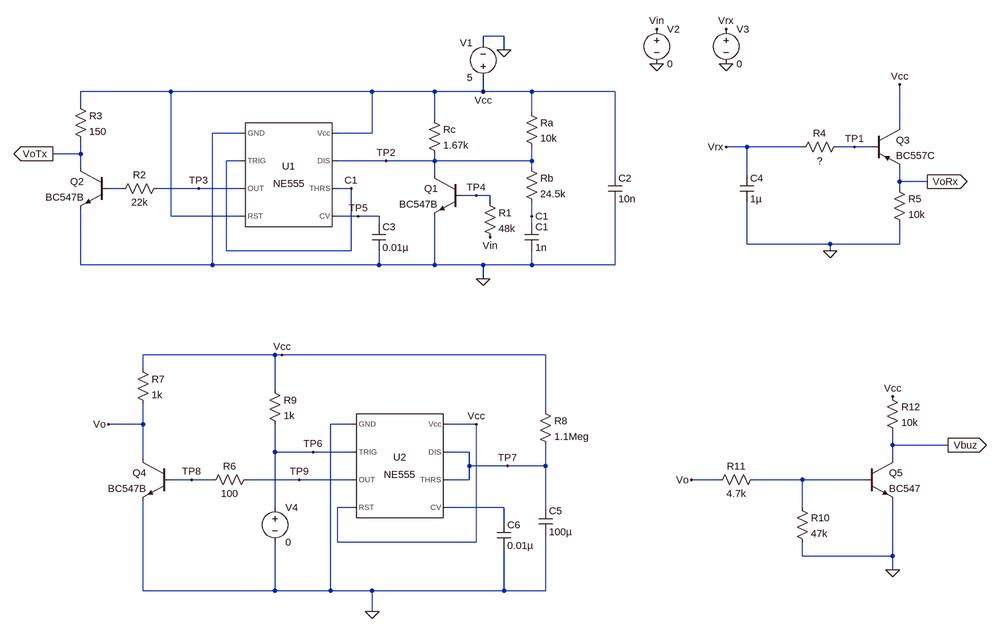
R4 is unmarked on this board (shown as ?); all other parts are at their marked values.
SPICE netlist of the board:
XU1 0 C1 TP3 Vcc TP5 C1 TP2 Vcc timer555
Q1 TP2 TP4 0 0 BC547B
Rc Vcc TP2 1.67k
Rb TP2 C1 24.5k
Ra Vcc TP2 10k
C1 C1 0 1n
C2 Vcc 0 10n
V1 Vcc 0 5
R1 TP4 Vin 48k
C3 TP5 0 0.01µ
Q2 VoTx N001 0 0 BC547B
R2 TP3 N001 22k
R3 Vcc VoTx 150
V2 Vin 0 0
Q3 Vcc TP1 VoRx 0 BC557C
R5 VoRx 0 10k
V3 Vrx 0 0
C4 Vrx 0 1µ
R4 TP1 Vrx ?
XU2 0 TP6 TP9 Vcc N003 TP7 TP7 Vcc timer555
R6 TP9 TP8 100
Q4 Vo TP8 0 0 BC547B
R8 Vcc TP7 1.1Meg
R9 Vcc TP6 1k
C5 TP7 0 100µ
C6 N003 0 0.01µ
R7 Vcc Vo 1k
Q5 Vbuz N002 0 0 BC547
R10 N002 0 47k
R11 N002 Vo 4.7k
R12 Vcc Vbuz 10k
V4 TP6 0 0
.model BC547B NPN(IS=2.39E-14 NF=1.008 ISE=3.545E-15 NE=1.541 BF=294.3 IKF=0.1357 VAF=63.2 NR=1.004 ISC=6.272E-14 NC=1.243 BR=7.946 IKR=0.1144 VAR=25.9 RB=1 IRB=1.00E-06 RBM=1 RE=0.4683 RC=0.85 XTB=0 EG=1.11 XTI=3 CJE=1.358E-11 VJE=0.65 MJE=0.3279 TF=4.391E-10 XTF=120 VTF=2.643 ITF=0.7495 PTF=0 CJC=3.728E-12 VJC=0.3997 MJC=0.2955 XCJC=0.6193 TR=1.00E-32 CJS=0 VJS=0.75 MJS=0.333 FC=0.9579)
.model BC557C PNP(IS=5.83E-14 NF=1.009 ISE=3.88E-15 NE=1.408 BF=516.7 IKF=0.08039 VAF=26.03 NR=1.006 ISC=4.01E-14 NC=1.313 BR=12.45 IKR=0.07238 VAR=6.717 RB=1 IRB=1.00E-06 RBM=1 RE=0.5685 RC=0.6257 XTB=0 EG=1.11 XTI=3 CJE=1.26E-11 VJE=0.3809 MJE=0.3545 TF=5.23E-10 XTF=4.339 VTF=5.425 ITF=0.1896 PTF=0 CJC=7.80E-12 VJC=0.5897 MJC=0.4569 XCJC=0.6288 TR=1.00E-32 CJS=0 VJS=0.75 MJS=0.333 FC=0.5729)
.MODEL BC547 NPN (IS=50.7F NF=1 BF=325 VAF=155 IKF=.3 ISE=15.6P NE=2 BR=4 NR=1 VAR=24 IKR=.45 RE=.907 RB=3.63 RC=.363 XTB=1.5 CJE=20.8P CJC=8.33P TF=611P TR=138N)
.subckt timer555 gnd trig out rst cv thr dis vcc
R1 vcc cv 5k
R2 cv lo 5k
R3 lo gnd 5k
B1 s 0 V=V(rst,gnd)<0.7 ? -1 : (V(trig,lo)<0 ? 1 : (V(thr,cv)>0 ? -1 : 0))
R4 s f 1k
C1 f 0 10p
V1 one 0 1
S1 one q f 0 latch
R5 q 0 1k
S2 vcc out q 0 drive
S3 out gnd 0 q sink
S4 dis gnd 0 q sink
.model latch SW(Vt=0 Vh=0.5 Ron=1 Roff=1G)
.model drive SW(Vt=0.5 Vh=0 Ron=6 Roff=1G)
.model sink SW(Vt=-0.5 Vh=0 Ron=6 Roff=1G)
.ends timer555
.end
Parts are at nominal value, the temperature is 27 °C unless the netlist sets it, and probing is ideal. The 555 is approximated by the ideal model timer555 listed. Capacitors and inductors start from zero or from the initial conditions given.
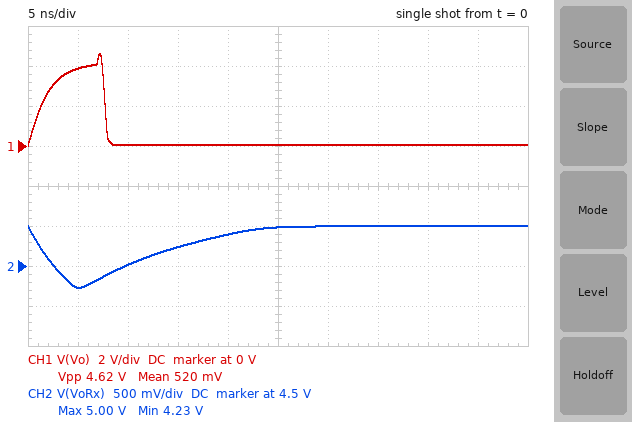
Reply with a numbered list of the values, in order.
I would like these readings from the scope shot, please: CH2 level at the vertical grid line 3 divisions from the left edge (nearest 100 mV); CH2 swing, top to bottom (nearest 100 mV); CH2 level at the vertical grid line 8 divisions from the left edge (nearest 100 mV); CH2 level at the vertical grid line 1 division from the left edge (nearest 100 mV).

1. 4.7 V
2. 800 mV
3. 5.0 V
4. 4.2 V
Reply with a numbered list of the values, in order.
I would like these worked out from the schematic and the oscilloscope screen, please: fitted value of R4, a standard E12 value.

1. 4.7 kΩ
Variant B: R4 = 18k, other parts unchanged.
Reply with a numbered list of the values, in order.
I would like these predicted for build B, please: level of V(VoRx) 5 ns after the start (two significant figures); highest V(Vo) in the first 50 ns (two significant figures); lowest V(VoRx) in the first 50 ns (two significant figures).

1. 4.4 V
2. 4.6 V
3. 4.0 V
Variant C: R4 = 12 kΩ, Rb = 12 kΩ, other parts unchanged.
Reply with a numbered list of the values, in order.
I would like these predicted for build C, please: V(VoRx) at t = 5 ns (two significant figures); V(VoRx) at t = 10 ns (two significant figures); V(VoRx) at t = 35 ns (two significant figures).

1. 4.4 V
2. 4.1 V
3. 4.7 V
